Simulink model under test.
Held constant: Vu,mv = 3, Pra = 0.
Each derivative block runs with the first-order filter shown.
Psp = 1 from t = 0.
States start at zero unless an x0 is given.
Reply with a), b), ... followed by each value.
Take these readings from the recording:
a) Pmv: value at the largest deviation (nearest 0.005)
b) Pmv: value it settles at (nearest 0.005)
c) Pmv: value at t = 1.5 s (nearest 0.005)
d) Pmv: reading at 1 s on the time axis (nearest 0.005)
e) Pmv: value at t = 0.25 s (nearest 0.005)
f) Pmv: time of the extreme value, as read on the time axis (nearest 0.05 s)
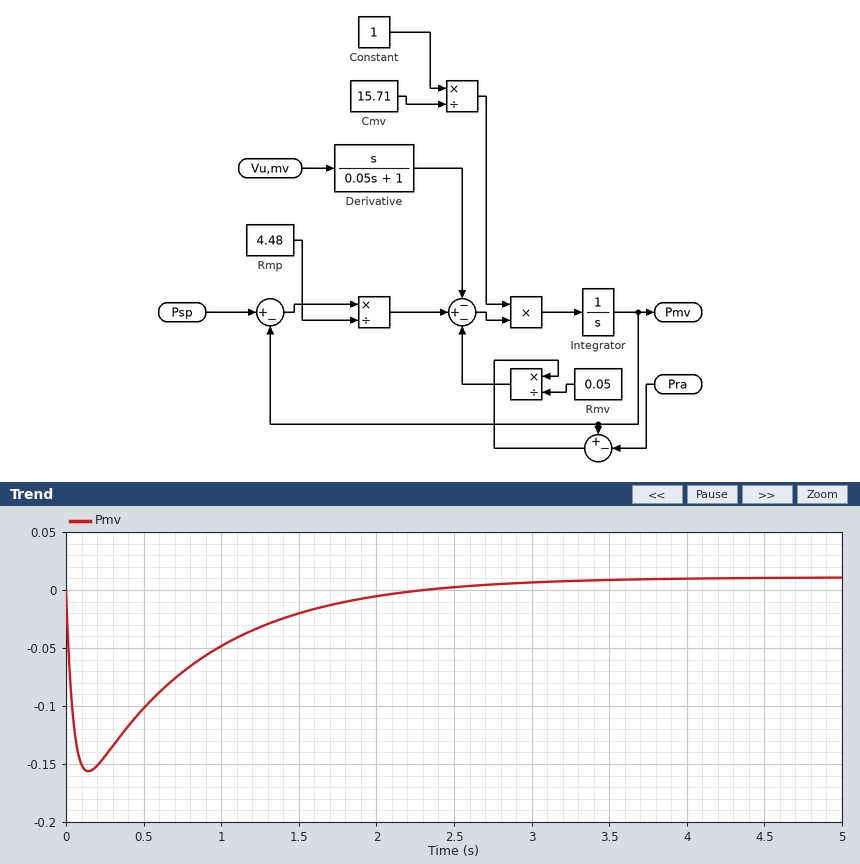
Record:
a) -0.155
b) 0.010
c) -0.020
d) -0.050
e) -0.145
f) 0.15 s
